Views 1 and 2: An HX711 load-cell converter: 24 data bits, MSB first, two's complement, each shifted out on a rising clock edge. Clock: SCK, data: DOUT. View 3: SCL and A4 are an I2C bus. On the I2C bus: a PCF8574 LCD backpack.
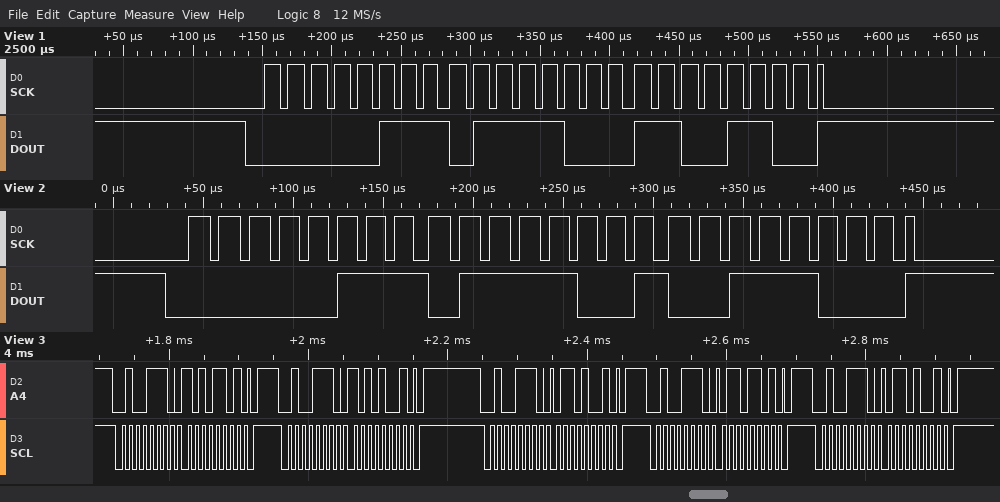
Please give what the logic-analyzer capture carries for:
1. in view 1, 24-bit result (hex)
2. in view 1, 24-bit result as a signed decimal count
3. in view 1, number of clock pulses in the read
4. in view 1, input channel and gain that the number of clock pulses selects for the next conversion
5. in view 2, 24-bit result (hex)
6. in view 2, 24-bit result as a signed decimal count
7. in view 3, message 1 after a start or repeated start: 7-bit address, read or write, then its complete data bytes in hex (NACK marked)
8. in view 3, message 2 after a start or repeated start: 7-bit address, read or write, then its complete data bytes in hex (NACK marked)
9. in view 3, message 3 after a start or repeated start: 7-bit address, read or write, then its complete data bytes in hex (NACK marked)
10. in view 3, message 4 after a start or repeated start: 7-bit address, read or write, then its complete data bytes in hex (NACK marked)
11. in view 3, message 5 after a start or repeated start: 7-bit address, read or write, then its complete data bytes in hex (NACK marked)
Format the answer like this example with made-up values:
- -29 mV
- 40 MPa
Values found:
- 0x0778CC
- 489676
- 25
- channel A, gain 128
- 0x077938
- 489784
- 0x27 write: AD
- 0x27 write: A9
- 0x27 write: 69
- 0x27 write: 6D
- 0x27 write: 69
